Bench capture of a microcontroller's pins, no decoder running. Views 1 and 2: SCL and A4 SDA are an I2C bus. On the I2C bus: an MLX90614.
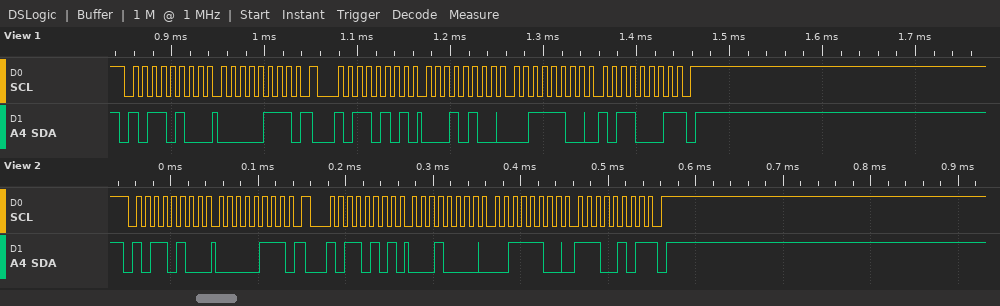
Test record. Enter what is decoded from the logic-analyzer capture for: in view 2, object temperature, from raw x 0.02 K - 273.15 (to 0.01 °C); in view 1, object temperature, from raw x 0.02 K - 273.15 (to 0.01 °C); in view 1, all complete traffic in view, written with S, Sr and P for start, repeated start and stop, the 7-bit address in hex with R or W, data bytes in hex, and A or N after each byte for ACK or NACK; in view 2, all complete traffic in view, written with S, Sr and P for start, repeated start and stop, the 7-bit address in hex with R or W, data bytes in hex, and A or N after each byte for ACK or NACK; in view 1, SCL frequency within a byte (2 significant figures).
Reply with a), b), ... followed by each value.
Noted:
a) 34.37 °C
b) 34.45 °C
c) S 5AW A 07 A Sr 5AR A 14 A 3C A B1 N P
d) S 5AW A 07 A Sr 5AR A 10 A 3C A E5 N P
e) 100 kHz
